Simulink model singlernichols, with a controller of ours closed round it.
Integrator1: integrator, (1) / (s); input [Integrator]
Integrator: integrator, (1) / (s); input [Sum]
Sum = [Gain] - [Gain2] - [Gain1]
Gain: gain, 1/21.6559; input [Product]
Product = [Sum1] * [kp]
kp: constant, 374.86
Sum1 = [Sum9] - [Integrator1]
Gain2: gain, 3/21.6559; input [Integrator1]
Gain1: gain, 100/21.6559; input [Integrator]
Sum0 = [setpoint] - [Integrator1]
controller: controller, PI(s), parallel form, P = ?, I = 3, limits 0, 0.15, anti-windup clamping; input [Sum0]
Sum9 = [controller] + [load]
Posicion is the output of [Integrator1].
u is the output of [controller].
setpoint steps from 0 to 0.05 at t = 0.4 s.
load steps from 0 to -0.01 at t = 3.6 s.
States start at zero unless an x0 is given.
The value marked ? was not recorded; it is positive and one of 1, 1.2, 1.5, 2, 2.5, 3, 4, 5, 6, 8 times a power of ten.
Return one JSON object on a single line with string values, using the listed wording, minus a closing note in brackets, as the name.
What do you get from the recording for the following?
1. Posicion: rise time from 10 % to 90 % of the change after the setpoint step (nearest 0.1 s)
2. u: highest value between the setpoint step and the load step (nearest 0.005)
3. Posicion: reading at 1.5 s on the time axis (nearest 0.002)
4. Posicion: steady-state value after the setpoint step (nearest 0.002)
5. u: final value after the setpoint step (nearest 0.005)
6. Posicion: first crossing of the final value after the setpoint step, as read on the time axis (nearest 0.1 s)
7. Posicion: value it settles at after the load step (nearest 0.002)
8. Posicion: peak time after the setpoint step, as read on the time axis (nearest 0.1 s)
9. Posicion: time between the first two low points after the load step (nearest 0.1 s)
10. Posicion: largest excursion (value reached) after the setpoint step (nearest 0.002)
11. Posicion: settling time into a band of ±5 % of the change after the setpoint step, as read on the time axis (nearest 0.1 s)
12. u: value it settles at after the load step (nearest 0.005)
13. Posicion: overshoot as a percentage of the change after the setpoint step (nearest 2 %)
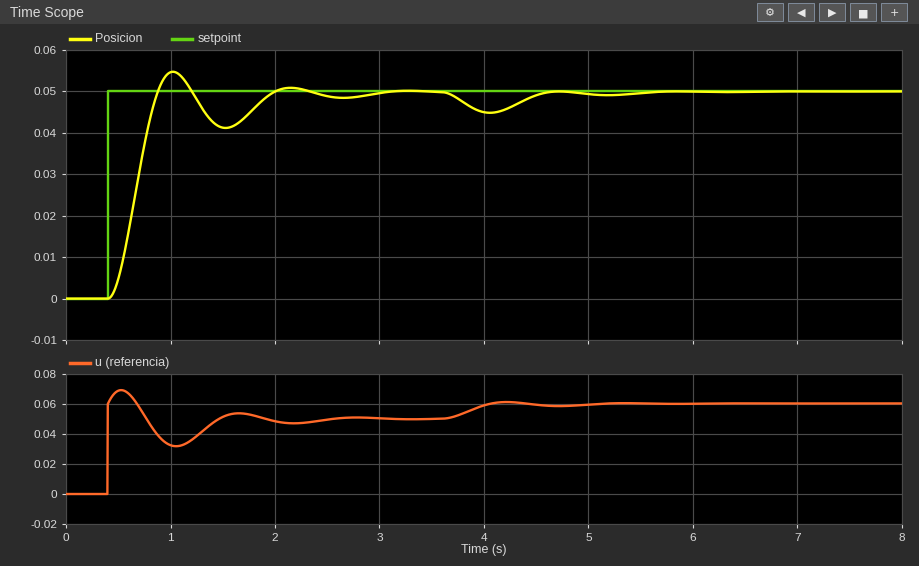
{"Posicion: rise time from 10 % to 90 % of the change after the setpoint step": "0.3 s", "u: highest value between the setpoint step and the load step": "0.070", "Posicion: reading at 1.5 s on the time axis": "0.042", "Posicion: steady-state value after the setpoint step": "0.050", "u: final value after the setpoint step": "0.050", "Posicion: first crossing of the final value after the setpoint step, as read on the time axis": "0.9 s", "Posicion: value it settles at after the load step": "0.050", "Posicion: peak time after the setpoint step, as read on the time axis": "1.0 s", "Posicion: time between the first two low points after the load step": "1.1 s", "Posicion: largest excursion (value reached) after the setpoint step": "0.054", "Posicion: settling time into a band of ±5 % of the change after the setpoint step, as read on the time axis": "1.9 s", "u: value it settles at after the load step": "0.060", "Posicion: overshoot as a percentage of the change after the setpoint step": "10 %"}
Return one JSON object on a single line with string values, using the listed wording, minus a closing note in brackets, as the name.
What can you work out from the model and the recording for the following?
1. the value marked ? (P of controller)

{"the value marked ?": "1.2"}
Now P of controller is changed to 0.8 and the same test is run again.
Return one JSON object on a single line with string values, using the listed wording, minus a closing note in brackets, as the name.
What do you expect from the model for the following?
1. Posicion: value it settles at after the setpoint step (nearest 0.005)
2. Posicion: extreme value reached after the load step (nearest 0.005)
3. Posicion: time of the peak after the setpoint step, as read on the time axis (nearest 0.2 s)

{"Posicion: value it settles at after the setpoint step": "0.050", "Posicion: extreme value reached after the load step": "0.045", "Posicion: time of the peak after the setpoint step, as read on the time axis": "1.2 s"}
